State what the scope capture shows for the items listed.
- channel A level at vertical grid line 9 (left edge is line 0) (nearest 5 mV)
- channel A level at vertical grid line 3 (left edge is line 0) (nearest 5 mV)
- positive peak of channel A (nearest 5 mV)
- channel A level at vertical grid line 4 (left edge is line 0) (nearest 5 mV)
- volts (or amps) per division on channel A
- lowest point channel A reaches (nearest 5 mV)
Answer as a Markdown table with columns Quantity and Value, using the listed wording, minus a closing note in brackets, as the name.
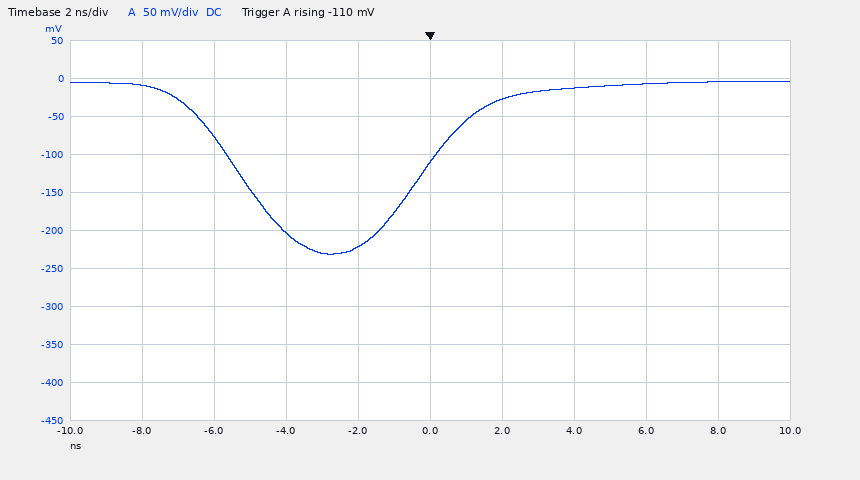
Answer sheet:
| Quantity | Value |
|---|---|
| channel A level at vertical grid line 9 (left edge is line 0) | -5 mV |
| channel A level at vertical grid line 3 (left edge is line 0) | -205 mV |
| positive peak of channel A | -5 mV |
| channel A level at vertical grid line 4 (left edge is line 0) | -220 mV |
| volts (or amps) per division on channel A | 50 mV |
| lowest point channel A reaches | -230 mV |
